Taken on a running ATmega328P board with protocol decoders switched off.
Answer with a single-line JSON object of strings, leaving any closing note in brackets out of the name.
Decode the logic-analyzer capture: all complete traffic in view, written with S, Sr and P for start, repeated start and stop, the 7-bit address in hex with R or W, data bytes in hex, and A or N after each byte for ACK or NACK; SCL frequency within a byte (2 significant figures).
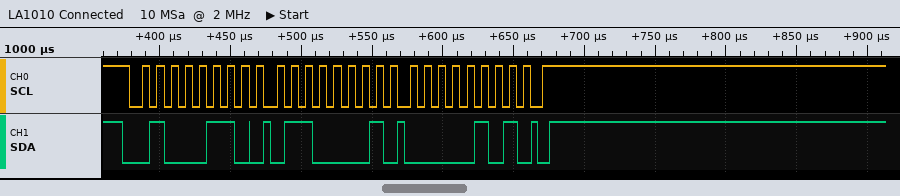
{"all complete traffic in view, written with S, Sr and P for start, repeated start and stop, the 7-bit address in hex with R or W, data bytes in hex, and A or N after each byte for ACK or NACK": "S 23W A 61 A 05 A P", "SCL frequency within a byte": "100 kHz"}
